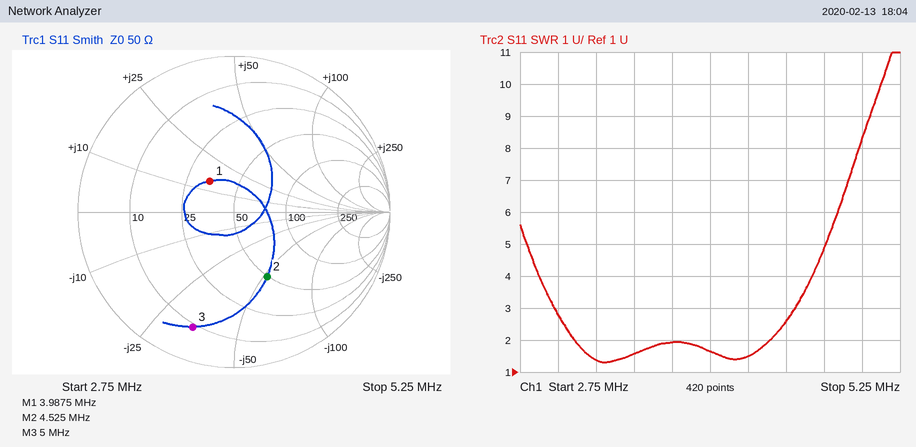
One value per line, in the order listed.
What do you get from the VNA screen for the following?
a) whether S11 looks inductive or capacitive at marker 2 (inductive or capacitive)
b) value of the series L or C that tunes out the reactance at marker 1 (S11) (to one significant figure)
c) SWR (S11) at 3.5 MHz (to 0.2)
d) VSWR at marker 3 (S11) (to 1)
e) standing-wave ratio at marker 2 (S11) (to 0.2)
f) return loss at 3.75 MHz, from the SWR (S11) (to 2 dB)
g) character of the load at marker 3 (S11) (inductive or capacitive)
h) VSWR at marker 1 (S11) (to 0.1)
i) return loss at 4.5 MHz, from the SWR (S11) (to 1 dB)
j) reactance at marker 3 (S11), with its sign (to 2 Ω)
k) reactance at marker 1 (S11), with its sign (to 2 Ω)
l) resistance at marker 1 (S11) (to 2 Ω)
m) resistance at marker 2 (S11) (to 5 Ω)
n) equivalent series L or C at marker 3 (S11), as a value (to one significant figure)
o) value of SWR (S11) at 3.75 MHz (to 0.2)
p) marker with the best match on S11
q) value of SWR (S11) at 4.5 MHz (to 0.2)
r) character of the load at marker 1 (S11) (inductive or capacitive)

capacitive
3 nF
1.6
8
2.8
10 dB
capacitive
1.7
7 dB
-34 Ω
+14 Ω
34 Ω
50 Ω
900 pF
2.0
marker 1
2.6
inductive
